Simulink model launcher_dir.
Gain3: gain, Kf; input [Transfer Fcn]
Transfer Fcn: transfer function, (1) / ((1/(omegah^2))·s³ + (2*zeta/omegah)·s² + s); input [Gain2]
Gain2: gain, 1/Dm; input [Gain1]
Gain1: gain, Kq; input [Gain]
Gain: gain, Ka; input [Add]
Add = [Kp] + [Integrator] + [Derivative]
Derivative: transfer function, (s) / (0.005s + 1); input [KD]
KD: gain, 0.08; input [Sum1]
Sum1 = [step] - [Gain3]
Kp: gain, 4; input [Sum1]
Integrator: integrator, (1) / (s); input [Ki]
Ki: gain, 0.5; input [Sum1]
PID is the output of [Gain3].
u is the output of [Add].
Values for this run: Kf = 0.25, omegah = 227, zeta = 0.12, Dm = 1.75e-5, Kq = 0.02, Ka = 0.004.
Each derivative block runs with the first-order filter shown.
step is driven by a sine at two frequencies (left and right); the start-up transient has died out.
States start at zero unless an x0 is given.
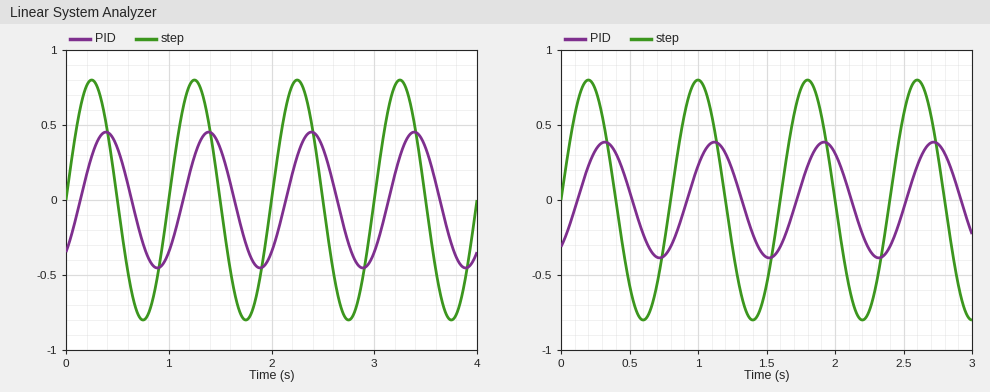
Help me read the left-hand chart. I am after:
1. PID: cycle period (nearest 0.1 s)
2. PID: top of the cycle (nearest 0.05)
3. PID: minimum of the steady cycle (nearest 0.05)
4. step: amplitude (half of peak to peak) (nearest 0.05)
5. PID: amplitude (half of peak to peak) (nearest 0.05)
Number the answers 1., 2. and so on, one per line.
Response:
1. 1.0 s
2. 0.45
3. -0.45
4. 0.80
5. 0.45
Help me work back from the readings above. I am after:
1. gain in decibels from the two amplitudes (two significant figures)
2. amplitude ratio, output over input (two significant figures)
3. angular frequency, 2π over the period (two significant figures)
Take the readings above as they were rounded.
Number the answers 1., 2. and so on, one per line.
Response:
1. -5.0 dB
2. 0.56
3. 6.3 rad/s
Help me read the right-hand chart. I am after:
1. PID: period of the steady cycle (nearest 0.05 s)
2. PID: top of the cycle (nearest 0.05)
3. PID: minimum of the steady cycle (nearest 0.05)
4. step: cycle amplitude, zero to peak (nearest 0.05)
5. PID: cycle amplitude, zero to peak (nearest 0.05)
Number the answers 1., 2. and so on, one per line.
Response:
1. 0.80 s
2. 0.40
3. -0.40
4. 0.80
5. 0.40
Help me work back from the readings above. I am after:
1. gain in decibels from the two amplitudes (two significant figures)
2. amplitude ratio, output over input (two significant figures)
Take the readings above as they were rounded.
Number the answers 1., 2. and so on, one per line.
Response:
1. -6.0 dB
2. 0.50
